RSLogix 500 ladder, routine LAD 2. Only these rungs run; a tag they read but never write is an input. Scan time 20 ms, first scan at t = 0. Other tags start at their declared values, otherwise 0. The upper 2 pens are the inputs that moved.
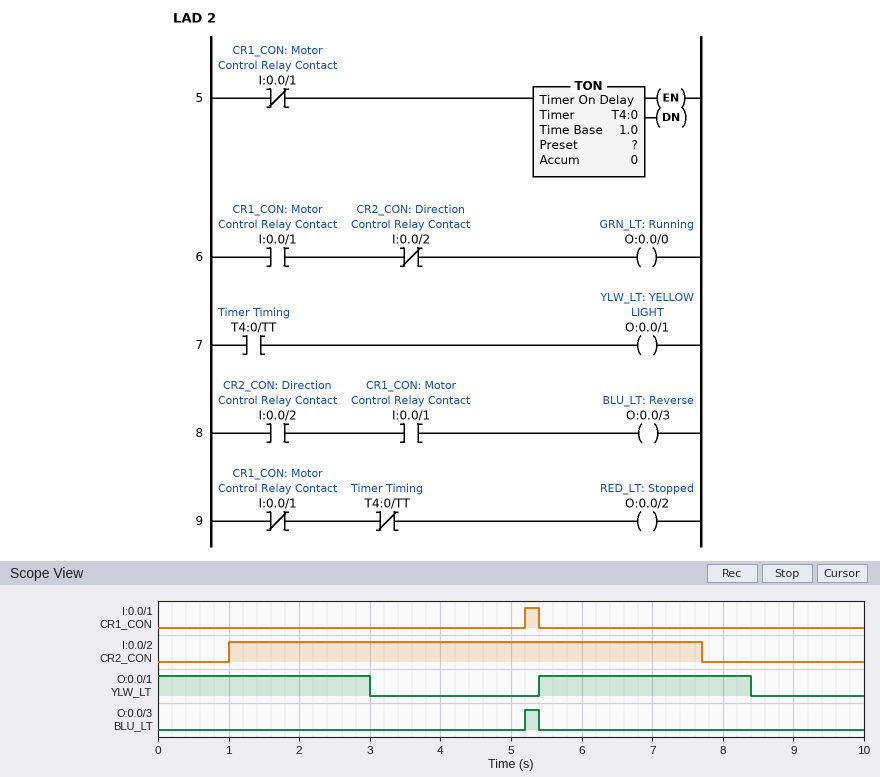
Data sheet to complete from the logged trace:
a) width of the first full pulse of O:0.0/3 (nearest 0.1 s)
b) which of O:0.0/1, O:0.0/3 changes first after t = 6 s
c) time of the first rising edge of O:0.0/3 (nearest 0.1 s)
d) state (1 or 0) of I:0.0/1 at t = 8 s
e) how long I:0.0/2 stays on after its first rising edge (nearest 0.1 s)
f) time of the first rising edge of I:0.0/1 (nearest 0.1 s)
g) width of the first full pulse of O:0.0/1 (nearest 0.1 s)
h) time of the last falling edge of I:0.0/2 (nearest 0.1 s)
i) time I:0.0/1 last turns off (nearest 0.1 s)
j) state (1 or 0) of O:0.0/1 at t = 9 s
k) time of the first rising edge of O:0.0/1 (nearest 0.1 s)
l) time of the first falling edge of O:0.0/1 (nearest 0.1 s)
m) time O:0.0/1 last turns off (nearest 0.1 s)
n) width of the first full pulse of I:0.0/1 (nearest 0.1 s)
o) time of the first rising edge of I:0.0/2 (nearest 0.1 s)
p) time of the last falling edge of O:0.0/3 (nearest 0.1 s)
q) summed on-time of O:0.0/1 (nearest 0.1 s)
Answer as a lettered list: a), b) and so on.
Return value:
a) 0.2 s
b) O:0.0/1
c) 5.2 s
d) 0
e) 6.7 s
f) 5.2 s
g) 3.0 s
h) 7.7 s
i) 5.4 s
j) 0
k) 5.4 s
l) 3.0 s
m) 8.4 s
n) 0.2 s
o) 1.0 s
p) 5.4 s
q) 6.0 s
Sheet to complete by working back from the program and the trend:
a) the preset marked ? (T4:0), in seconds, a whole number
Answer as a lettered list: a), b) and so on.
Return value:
a) 3 s
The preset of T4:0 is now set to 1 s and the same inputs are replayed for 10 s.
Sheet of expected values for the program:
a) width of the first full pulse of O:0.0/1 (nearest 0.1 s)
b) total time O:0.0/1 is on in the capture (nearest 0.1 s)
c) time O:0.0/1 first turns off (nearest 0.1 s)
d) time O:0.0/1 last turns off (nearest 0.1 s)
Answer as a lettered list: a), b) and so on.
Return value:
a) 1.0 s
b) 2.0 s
c) 1.0 s
d) 6.4 s
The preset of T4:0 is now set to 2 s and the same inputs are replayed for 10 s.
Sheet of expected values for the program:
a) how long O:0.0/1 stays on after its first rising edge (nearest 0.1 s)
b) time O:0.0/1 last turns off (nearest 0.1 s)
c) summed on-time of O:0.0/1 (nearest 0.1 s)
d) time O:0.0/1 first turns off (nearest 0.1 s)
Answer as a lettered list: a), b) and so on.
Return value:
a) 2.0 s
b) 7.4 s
c) 4.0 s
d) 2.0 s
